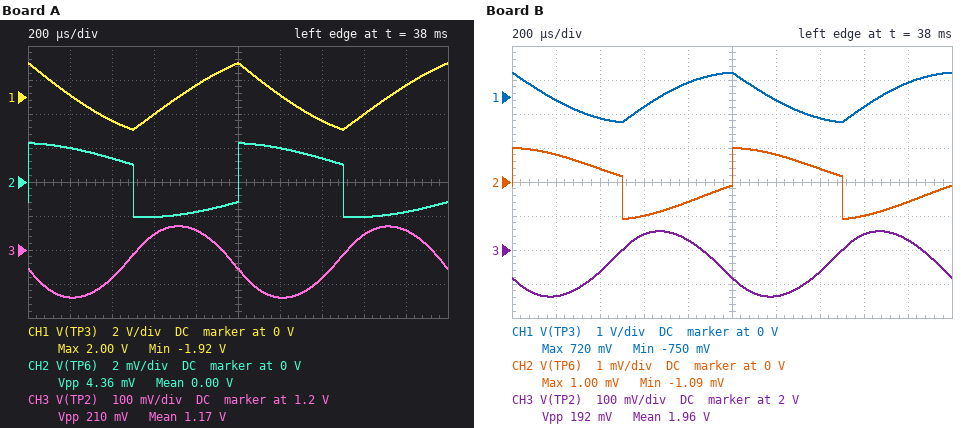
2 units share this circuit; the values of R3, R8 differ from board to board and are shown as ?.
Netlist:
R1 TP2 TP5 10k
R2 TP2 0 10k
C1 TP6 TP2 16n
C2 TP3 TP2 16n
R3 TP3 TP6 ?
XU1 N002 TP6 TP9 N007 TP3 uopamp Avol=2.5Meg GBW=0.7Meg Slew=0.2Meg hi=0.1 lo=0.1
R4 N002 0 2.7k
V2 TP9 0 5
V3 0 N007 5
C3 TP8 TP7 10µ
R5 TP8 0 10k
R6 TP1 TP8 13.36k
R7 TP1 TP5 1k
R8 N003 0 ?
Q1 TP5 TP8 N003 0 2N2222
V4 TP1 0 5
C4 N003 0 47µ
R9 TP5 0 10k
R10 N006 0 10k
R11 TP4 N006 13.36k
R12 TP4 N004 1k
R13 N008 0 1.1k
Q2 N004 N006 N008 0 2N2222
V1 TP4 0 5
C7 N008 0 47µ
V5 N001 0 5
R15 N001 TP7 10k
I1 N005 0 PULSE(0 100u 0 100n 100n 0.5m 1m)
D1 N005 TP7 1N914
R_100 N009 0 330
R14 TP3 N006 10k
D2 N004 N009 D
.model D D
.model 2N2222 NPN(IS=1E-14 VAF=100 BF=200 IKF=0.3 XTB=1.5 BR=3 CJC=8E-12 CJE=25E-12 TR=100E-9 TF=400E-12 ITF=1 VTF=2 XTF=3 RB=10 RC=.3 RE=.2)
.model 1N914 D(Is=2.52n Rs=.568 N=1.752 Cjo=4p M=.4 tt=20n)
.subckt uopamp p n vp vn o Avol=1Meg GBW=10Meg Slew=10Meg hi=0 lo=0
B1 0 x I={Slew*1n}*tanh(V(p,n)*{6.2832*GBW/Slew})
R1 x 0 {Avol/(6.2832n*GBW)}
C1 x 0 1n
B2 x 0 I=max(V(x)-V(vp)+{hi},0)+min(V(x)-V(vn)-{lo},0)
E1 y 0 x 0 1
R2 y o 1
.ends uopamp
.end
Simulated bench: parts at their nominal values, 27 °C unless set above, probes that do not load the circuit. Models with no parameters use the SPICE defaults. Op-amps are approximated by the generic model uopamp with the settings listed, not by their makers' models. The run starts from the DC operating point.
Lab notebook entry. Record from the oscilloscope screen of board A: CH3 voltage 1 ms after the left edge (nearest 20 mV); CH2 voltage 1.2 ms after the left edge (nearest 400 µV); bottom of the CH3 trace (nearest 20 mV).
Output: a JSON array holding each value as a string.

["1.14 V", "2.0 mV", "1.06 V"]
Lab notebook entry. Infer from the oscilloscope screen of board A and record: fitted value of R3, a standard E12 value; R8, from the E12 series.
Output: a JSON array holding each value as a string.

["150 kΩ", "470 Ω"]
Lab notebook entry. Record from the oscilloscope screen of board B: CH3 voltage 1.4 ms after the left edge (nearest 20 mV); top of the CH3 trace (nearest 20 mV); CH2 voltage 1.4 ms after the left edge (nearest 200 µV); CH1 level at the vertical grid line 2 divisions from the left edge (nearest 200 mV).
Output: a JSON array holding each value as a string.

["1.94 V", "2.06 V", "400 µV", "-600 mV"]
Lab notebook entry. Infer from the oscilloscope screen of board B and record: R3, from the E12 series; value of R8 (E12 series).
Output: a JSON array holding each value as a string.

["68 kΩ", "3.3 kΩ"]
